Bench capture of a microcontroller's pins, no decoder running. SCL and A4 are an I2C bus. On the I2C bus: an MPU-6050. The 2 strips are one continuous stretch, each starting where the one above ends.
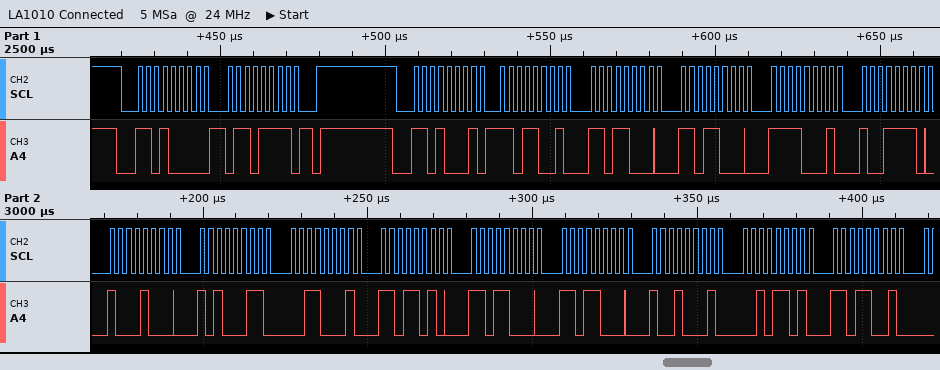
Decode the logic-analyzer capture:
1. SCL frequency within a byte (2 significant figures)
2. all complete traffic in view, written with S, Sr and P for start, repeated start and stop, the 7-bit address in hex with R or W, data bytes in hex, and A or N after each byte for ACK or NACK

400 kHz
S 68W A 6F A P S 68R A D9 A D8 A D8 A F1 A 9E A 88 A A3 A 31 A DA A D8 A D8 A 91 A 2D A D9 A
